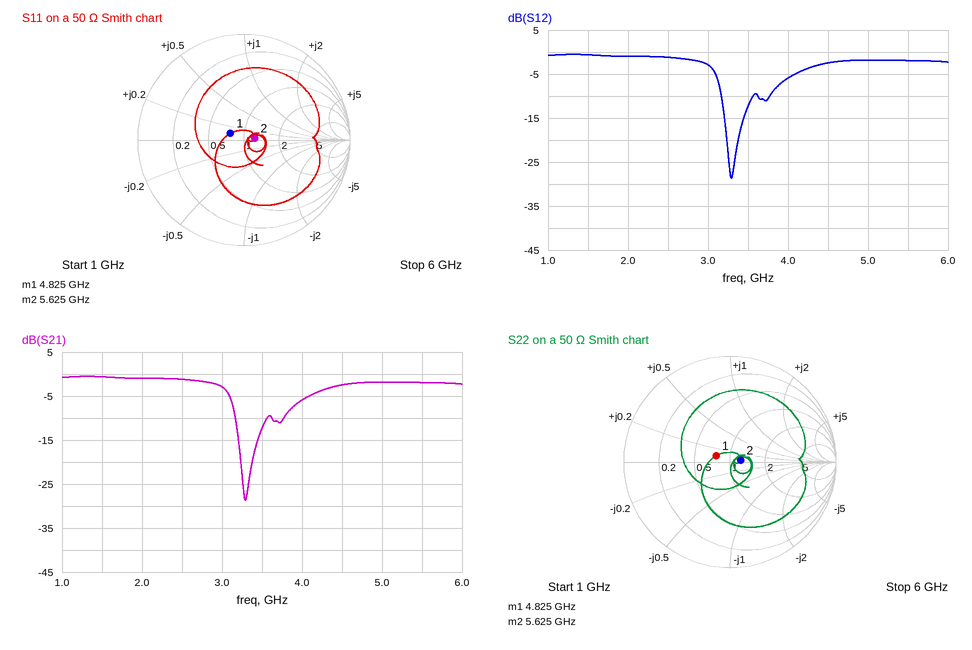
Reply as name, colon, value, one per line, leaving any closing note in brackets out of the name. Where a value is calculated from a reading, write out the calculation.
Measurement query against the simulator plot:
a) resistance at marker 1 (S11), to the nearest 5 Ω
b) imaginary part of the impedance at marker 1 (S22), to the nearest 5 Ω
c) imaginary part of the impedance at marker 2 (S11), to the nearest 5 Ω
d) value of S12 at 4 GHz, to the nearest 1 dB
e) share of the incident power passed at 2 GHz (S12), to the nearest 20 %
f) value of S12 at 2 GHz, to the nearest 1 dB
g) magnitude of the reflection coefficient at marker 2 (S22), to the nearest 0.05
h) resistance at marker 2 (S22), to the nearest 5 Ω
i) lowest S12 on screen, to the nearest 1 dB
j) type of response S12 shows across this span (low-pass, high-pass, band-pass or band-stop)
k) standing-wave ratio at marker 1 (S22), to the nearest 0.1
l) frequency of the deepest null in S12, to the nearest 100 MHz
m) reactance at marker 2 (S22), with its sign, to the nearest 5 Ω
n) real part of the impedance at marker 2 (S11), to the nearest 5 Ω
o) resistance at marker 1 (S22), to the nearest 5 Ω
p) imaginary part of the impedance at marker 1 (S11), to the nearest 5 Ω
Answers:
resistance at marker 1 (S11), to the nearest 5 Ω: 40 Ω
imaginary part of the impedance at marker 1 (S22), to the nearest 5 Ω: +5 Ω
imaginary part of the impedance at marker 2 (S11), to the nearest 5 Ω: 0 Ω
value of S12 at 4 GHz, to the nearest 1 dB: -6 dB
share of the incident power passed at 2 GHz (S12), to the nearest 20 %: 10^(-1/10) ≈ 79.4 %, so 80 % to the nearest 20 %
value of S12 at 2 GHz, to the nearest 1 dB: -1 dB
magnitude of the reflection coefficient at marker 2 (S22), to the nearest 0.05: 0.10
resistance at marker 2 (S22), to the nearest 5 Ω: 60 Ω
lowest S12 on screen, to the nearest 1 dB: -29 dB
type of response S12 shows across this span: band-stop
standing-wave ratio at marker 1 (S22), to the nearest 0.1: 1.3
frequency of the deepest null in S12, to the nearest 100 MHz: 3.3 GHz
reactance at marker 2 (S22), with its sign, to the nearest 5 Ω: 0 Ω
real part of the impedance at marker 2 (S11), to the nearest 5 Ω: 60 Ω
resistance at marker 1 (S22), to the nearest 5 Ω: 40 Ω
imaginary part of the impedance at marker 1 (S11), to the nearest 5 Ω: +5 Ω
